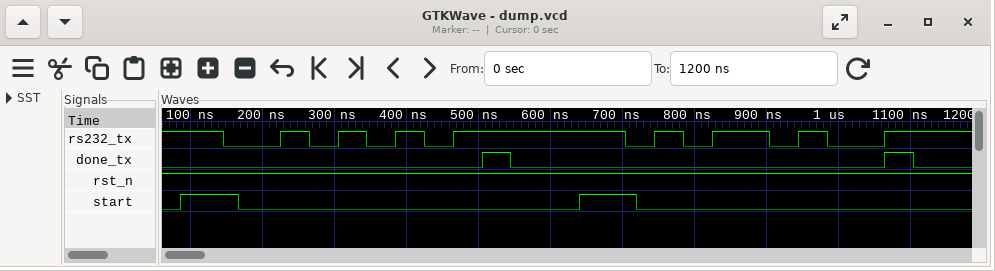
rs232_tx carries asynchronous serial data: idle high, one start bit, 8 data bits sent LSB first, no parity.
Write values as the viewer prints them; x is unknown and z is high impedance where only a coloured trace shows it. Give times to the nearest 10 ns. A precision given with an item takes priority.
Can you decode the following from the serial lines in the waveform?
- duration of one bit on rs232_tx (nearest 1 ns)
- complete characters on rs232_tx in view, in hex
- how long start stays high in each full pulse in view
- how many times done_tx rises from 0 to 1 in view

40 ns
AA, 2D
80 ns, 80 ns
2
